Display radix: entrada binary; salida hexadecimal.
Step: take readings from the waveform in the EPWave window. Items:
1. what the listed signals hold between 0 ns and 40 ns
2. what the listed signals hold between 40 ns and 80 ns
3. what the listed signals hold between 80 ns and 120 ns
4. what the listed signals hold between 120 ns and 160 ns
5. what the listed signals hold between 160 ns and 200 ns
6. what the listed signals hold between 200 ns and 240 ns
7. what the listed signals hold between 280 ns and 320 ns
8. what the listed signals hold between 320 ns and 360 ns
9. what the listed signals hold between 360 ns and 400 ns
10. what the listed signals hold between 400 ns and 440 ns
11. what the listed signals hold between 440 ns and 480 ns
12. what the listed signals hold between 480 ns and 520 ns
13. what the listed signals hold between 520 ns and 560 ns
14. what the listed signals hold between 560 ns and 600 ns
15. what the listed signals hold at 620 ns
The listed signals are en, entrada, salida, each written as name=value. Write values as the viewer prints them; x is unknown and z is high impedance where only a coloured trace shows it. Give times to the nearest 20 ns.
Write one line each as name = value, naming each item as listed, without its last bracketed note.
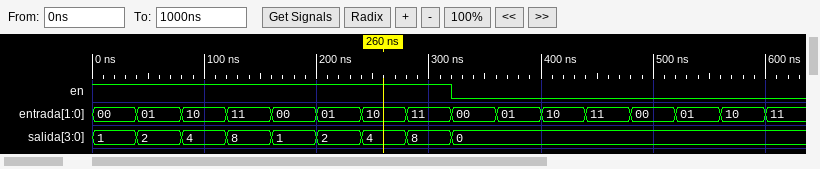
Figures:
what the listed signals hold between 0 ns and 40 ns = en=1, entrada=00, salida=1
what the listed signals hold between 40 ns and 80 ns = en=1, entrada=01, salida=2
what the listed signals hold between 80 ns and 120 ns = en=1, entrada=10, salida=4
what the listed signals hold between 120 ns and 160 ns = en=1, entrada=11, salida=8
what the listed signals hold between 160 ns and 200 ns = en=1, entrada=00, salida=1
what the listed signals hold between 200 ns and 240 ns = en=1, entrada=01, salida=2
what the listed signals hold between 280 ns and 320 ns = en=1, entrada=11, salida=8
what the listed signals hold between 320 ns and 360 ns = en=0, entrada=00, salida=0
what the listed signals hold between 360 ns and 400 ns = en=0, entrada=01, salida=0
what the listed signals hold between 400 ns and 440 ns = en=0, entrada=10, salida=0
what the listed signals hold between 440 ns and 480 ns = en=0, entrada=11, salida=0
what the listed signals hold between 480 ns and 520 ns = en=0, entrada=00, salida=0
what the listed signals hold between 520 ns and 560 ns = en=0, entrada=01, salida=0
what the listed signals hold between 560 ns and 600 ns = en=0, entrada=10, salida=0
what the listed signals hold at 620 ns = en=0, entrada=11, salida=0
